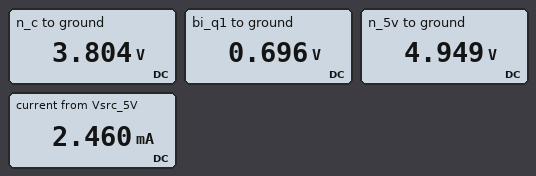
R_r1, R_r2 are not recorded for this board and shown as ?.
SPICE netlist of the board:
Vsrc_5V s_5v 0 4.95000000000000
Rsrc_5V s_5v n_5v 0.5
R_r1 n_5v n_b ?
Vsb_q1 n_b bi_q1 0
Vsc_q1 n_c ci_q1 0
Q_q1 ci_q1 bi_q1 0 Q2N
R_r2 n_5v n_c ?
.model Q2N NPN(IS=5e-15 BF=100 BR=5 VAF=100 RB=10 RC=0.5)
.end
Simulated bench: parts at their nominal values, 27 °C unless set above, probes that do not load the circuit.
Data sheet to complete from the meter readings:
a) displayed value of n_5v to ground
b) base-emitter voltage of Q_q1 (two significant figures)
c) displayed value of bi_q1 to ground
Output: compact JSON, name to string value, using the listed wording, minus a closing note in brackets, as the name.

{"displayed value of n_5v to ground": "4.949 V", "base-emitter voltage of Q_q1": "700 mV", "displayed value of bi_q1 to ground": "0.696 V"}
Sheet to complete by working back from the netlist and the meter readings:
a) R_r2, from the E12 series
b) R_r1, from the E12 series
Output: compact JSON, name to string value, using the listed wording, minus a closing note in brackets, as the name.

{"R_r2, from the E12 series": "470 Ω", "R_r1, from the E12 series": "180 kΩ"}
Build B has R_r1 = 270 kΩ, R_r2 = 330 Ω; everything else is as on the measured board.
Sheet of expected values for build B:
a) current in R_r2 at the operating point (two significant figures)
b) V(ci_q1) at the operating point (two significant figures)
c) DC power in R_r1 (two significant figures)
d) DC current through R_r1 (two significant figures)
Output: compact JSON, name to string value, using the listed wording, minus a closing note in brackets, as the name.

{"current in R_r2 at the operating point": "1.6 mA", "V(ci_q1) at the operating point": "4.4 V", "DC power in R_r1": "67 µW", "DC current through R_r1": "16 µA"}
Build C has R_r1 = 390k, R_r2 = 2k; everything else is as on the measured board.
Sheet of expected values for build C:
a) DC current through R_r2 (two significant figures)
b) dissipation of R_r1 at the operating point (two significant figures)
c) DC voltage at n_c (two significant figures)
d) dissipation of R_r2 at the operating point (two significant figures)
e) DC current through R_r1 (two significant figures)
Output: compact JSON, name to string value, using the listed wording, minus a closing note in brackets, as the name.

{"DC current through R_r2": "1.1 mA", "dissipation of R_r1 at the operating point": "47 µW", "DC voltage at n_c": "2.7 V", "dissipation of R_r2 at the operating point": "2.5 mW", "DC current through R_r1": "11 µA"}
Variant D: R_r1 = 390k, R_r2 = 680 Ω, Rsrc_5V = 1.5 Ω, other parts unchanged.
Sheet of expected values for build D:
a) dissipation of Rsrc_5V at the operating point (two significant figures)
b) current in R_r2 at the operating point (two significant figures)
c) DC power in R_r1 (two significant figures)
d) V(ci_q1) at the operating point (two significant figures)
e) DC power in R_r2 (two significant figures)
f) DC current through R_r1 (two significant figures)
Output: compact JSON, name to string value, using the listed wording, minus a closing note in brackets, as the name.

{"dissipation of Rsrc_5V at the operating point": "2.0 µW", "current in R_r2 at the operating point": "1.1 mA", "DC power in R_r1": "47 µW", "V(ci_q1) at the operating point": "4.2 V", "DC power in R_r2": "870 µW", "DC current through R_r1": "11 µA"}
